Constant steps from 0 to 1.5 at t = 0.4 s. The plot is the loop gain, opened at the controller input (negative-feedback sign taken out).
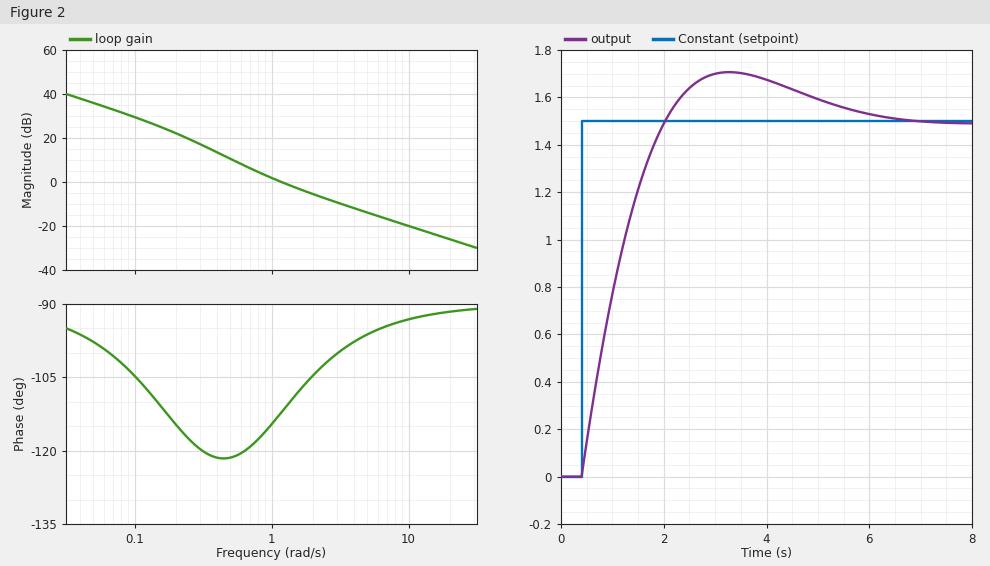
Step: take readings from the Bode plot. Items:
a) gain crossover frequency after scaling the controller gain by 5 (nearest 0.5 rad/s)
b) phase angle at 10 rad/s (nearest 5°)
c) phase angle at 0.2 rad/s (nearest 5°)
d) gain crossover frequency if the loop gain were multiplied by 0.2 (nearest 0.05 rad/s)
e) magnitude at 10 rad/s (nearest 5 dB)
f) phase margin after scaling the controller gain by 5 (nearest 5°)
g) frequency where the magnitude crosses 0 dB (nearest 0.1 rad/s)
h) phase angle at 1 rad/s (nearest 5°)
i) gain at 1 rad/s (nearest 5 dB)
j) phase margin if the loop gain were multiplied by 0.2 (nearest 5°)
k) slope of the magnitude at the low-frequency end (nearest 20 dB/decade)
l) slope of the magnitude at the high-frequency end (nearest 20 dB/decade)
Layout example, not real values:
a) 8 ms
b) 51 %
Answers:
a) 5.0 rad/s
b) -95°
c) -115°
d) 0.40 rad/s
e) -20 dB
f) 85°
g) 1.2 rad/s
h) -115°
i) 0 dB
j) 60°
k) -20 dB/decade
l) -20 dB/decade
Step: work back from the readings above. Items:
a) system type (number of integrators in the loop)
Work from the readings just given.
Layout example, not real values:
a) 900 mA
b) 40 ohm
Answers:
a) 1
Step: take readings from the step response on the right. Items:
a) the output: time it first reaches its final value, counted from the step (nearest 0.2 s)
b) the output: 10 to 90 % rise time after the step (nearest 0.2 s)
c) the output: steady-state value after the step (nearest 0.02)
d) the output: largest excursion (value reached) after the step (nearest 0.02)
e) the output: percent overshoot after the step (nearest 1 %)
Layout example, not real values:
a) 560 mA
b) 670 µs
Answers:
a) 1.6 s
b) 1.2 s
c) 1.50
d) 1.70
e) 14 %
